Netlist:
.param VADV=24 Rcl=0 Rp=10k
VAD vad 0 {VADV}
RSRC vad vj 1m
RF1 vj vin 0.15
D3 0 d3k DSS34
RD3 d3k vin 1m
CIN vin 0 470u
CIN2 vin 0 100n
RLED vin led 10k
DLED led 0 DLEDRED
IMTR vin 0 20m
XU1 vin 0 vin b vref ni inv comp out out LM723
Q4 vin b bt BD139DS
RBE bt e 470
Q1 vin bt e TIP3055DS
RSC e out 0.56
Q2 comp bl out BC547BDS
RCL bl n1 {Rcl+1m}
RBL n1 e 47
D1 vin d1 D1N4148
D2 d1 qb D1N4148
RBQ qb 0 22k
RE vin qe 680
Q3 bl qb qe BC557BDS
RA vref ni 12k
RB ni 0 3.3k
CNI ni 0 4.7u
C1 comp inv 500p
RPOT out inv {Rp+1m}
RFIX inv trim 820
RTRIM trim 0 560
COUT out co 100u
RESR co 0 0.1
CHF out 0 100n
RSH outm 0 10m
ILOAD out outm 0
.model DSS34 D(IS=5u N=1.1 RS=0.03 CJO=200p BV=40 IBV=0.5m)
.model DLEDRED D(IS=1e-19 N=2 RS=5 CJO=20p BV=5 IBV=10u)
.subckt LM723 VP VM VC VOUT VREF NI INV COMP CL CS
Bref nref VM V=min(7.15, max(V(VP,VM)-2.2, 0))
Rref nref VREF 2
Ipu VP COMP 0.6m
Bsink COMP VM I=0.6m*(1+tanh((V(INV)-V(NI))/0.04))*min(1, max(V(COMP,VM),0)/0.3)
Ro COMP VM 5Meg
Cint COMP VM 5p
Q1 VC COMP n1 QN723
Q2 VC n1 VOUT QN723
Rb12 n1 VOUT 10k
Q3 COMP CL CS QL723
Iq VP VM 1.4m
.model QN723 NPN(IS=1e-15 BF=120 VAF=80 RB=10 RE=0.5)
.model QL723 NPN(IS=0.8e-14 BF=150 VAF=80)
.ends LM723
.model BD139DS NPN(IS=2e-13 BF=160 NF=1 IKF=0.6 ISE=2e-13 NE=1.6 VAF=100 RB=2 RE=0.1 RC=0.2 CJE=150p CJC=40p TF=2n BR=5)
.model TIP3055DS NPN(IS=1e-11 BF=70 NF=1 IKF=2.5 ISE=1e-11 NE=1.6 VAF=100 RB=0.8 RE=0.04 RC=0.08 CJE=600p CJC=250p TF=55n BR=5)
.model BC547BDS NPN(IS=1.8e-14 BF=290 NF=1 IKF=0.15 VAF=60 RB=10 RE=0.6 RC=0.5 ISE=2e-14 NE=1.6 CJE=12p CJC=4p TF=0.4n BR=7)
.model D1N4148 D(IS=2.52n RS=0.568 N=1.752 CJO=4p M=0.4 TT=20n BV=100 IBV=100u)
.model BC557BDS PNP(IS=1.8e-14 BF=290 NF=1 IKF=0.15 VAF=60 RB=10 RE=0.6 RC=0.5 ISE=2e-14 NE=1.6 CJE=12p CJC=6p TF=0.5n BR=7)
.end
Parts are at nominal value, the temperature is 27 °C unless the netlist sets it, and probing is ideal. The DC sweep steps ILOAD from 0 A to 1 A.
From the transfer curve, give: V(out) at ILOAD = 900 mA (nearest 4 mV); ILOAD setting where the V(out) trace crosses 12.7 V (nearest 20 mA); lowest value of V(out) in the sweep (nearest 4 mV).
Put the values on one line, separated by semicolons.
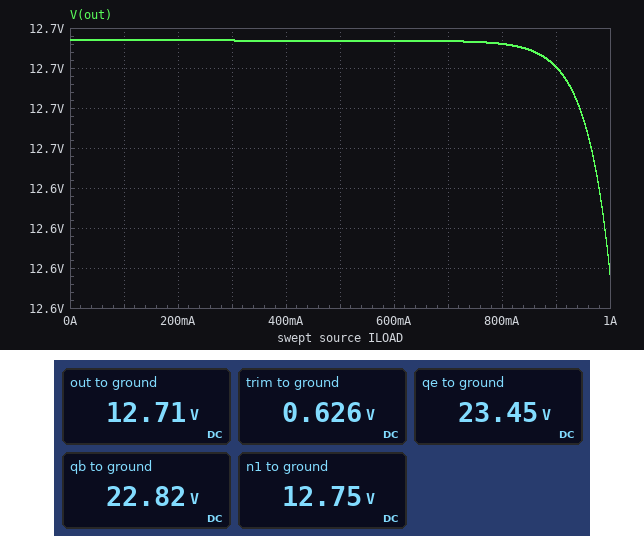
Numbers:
12.700 V; 900 mA; 12.596 V
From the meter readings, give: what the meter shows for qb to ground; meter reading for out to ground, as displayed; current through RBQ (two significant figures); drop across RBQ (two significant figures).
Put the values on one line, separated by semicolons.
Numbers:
22.82 V; 12.71 V; 1.0 mA; 23 V
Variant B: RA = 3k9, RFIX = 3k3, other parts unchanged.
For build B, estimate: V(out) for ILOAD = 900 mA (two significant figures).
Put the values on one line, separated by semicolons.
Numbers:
12 V
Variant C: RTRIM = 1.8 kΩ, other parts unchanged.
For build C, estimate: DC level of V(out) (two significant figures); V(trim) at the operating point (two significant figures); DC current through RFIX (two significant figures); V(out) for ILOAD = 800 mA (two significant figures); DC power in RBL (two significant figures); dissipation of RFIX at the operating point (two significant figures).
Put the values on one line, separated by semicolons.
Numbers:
7.5 V; 1.1 V; 590 µA; 7.4 V; 28 µW; 290 µW
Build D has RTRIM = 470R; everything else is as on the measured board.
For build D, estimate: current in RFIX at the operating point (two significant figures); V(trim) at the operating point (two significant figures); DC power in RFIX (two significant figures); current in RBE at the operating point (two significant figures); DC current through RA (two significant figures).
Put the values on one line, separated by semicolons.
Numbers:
1.2 mA; 560 mV; 1.2 mW; 400 µA; 470 µA
